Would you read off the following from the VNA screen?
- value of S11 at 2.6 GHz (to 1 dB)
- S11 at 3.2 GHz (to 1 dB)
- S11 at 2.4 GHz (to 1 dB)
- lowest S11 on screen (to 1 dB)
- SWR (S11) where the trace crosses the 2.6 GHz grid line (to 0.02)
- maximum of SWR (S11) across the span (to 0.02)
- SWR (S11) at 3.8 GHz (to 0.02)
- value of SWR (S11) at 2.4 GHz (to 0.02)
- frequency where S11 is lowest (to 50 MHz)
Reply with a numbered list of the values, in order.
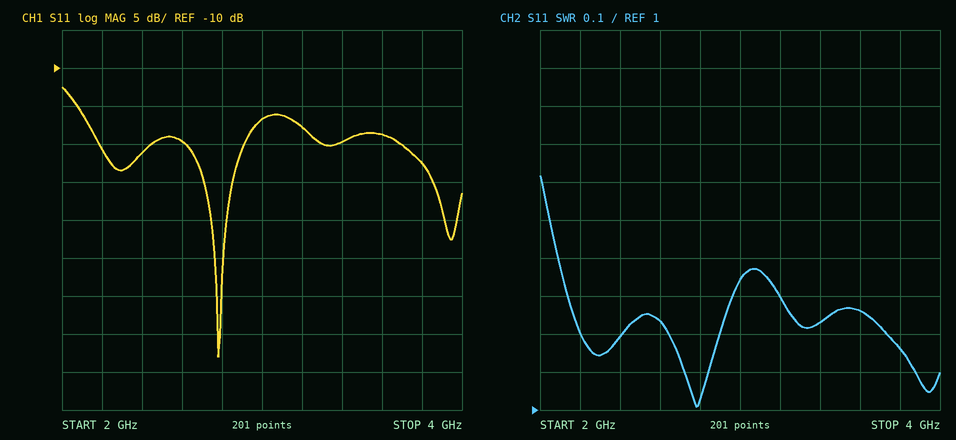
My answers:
1. -20 dB
2. -18 dB
3. -21 dB
4. -48 dB
5. 1.24
6. 1.62
7. 1.16
8. 1.20
9. 2.80 GHz
